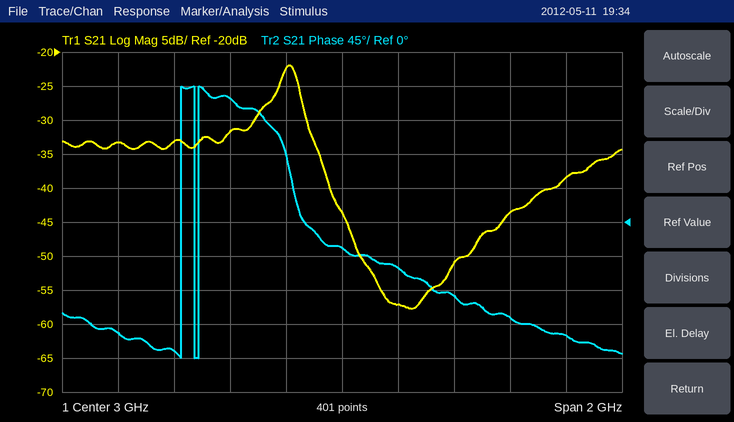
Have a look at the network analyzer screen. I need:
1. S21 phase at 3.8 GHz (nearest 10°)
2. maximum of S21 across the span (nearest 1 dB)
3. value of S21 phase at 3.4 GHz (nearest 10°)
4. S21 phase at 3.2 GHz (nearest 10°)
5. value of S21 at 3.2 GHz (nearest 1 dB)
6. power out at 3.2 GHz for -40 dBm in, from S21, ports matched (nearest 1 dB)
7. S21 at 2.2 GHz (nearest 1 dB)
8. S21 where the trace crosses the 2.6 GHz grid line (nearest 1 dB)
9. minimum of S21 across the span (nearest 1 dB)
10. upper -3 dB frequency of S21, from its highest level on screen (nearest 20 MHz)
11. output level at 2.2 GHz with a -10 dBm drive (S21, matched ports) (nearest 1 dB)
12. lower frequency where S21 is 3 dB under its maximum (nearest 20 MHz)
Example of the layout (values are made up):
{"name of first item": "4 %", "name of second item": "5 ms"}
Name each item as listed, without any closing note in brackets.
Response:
{"S21 phase at 3.8 GHz": "-150°", "maximum of S21 across the span": "-22 dB", "value of S21 phase at 3.4 GHz": "-100°", "S21 phase at 3.2 GHz": "-60°", "value of S21 at 3.2 GHz": "-57 dB", "power out at 3.2 GHz for -40 dBm in, from S21, ports matched": "-97 dBm", "S21 at 2.2 GHz": "-33 dB", "S21 where the trace crosses the 2.6 GHz grid line": "-32 dB", "minimum of S21 across the span": "-58 dB", "upper -3 dB frequency of S21, from its highest level on screen": "2.84 GHz", "output level at 2.2 GHz with a -10 dBm drive (S21, matched ports)": "-43 dBm", "lower frequency where S21 is 3 dB under its maximum": "2.78 GHz"}
